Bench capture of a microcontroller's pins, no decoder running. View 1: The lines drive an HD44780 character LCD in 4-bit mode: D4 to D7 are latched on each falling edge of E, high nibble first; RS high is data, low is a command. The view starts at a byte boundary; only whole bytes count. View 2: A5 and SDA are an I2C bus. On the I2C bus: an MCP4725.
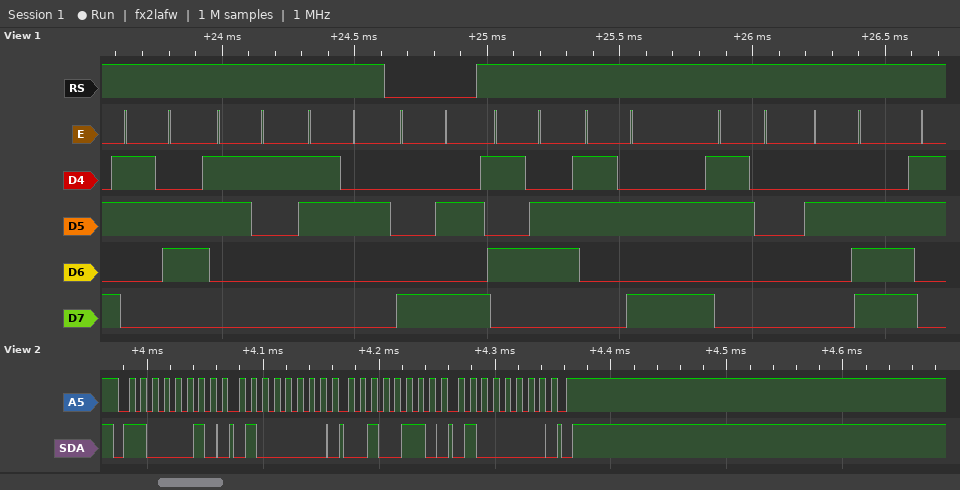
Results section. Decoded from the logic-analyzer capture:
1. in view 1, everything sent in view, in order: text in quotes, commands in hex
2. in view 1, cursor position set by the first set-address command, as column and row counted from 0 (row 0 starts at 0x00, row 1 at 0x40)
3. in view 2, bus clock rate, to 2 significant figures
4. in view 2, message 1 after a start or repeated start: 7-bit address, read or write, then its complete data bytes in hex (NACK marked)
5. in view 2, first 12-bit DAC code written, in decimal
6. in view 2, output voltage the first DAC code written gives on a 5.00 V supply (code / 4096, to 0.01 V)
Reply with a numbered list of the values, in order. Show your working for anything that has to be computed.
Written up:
1. "612" 0x8A "V:0."
2. column 10, row 0
3. 100 kHz
4. 0x61 write: 40 26 40
5. 612
6. 612 / 4096 x 5.00 V = 0.75 V
